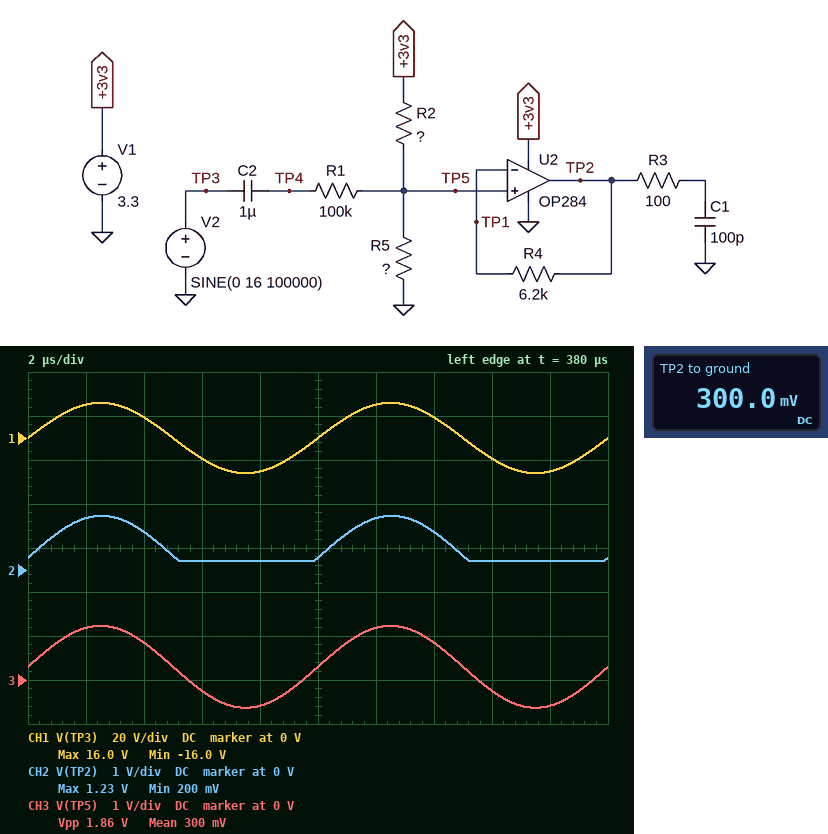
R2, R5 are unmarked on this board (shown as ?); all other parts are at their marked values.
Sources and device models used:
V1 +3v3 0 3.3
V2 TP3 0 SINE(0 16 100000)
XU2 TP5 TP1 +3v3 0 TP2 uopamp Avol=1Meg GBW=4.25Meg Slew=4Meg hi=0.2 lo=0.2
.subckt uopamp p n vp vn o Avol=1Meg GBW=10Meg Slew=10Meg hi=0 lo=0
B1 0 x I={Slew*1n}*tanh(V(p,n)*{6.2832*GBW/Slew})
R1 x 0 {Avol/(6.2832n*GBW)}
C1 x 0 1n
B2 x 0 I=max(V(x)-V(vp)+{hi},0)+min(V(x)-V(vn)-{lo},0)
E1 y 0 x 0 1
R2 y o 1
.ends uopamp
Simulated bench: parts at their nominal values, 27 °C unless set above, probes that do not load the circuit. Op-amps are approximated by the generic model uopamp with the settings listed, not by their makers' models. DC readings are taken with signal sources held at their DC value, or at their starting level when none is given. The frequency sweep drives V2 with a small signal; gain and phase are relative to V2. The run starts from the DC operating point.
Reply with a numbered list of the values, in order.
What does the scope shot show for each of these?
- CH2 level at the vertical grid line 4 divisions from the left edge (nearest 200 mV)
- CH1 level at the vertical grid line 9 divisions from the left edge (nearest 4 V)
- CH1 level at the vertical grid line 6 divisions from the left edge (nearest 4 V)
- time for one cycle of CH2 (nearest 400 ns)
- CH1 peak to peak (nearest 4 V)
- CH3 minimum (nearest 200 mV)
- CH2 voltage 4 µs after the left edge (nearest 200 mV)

1. 200 mV
2. -16 V
3. 16 V
4. 10.0 µs
5. 32 V
6. -600 mV
7. 800 mV
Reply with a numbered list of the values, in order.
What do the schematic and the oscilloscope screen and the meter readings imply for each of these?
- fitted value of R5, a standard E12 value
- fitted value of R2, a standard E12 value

1. 6.8 kΩ
2. 68 kΩ
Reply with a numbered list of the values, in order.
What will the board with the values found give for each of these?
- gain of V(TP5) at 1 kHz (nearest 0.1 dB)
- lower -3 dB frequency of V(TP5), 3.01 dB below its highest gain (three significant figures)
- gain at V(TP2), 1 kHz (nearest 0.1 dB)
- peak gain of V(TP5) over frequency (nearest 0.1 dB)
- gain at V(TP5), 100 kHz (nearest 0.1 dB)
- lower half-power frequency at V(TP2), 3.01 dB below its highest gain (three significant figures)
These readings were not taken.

1. -24.7 dB
2. 1.50 Hz
3. -24.7 dB
4. -24.7 dB
5. -24.7 dB
6. 1.50 Hz
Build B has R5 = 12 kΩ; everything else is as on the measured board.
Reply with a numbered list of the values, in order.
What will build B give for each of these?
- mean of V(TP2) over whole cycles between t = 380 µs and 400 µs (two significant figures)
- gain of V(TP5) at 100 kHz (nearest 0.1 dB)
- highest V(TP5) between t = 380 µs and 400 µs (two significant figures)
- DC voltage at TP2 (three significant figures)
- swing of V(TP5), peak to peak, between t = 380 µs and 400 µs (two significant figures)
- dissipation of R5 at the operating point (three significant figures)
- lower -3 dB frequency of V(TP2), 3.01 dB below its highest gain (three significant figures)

1. 830 mV
2. -20.7 dB
3. 2.0 V
4. 495 mV
5. 3.0 V
6. 20.4 µW
7. 1.44 Hz
